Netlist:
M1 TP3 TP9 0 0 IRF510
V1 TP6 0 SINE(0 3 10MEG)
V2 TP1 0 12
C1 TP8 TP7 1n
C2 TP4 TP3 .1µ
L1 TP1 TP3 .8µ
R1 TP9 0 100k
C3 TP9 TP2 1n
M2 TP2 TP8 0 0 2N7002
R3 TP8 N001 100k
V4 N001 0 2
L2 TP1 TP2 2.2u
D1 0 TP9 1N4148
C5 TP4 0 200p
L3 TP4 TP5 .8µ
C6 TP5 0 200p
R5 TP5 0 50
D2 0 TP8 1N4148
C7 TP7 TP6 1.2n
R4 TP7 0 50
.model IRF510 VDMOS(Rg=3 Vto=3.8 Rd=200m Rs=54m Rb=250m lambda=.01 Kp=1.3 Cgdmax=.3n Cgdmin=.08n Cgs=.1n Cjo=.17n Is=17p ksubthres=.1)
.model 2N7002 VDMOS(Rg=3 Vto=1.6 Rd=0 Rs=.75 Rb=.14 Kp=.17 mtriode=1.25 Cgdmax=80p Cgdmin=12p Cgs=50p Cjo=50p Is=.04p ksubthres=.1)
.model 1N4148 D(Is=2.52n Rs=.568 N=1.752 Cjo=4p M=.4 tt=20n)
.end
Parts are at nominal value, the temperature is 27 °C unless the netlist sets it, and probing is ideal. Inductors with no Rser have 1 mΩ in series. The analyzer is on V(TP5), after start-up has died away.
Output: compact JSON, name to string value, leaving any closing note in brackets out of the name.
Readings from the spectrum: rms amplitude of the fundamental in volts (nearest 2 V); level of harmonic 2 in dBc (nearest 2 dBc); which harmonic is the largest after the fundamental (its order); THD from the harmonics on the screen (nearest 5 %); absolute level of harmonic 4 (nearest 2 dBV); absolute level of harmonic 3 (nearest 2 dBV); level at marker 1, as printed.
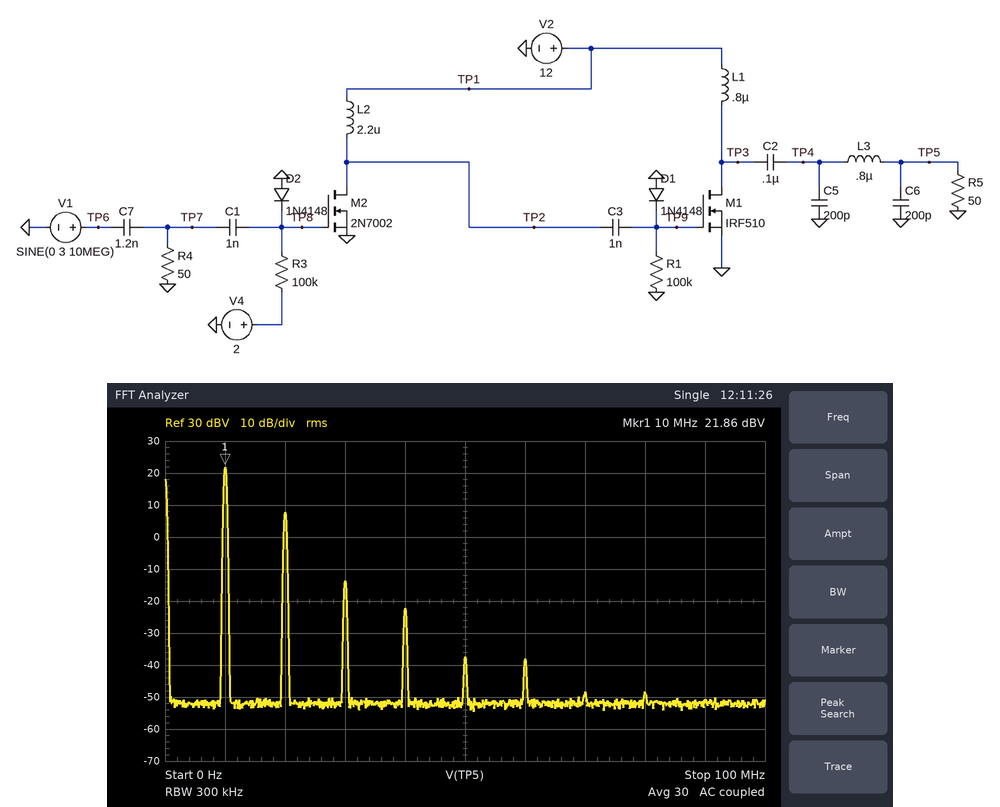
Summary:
{"rms amplitude of the fundamental in volts": "12 V", "level of harmonic 2 in dBc": "-14 dBc", "which harmonic is the largest after the fundamental": "2", "THD from the harmonics on the screen": "20 %", "absolute level of harmonic 4": "-22 dBV", "absolute level of harmonic 3": "-14 dBV", "level at marker 1, as printed": "21.86 dBV"}
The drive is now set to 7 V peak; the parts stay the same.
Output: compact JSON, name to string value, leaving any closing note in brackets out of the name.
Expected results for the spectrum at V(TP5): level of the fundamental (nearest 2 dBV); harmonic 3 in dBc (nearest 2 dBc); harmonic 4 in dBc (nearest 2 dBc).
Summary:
{"level of the fundamental": "22 dBV", "harmonic 3 in dBc": "-32 dBc", "harmonic 4 in dBc": "-46 dBc"}
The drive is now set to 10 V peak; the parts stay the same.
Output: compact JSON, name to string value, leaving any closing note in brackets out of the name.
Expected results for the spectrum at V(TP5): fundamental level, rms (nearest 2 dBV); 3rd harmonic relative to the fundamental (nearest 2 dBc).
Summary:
{"fundamental level, rms": "22 dBV", "3rd harmonic relative to the fundamental": "-32 dBc"}
